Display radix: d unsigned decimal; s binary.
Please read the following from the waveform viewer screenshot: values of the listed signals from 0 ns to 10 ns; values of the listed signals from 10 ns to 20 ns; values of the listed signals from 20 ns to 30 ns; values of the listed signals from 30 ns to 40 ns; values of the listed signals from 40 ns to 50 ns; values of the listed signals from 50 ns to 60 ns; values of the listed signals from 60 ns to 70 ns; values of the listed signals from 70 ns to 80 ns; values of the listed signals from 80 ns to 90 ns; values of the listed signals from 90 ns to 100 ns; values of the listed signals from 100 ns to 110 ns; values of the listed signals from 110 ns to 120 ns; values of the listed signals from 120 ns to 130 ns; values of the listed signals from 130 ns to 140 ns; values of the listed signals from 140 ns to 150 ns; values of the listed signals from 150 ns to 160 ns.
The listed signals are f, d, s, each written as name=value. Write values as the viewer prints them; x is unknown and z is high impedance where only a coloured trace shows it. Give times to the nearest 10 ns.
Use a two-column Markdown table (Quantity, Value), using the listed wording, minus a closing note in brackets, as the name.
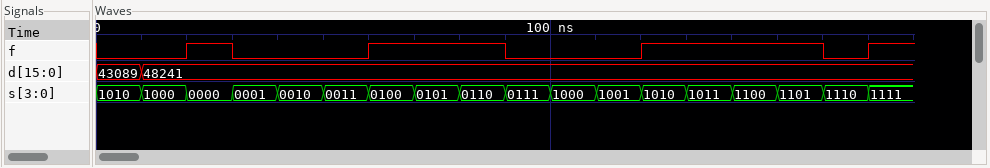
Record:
| Quantity | Value |
|---|---|
| values of the listed signals from 0 ns to 10 ns | f=0, d=43089, s=1010 |
| values of the listed signals from 10 ns to 20 ns | f=0, d=48241, s=1000 |
| values of the listed signals from 20 ns to 30 ns | f=1, d=48241, s=0000 |
| values of the listed signals from 30 ns to 40 ns | f=0, d=48241, s=0001 |
| values of the listed signals from 40 ns to 50 ns | f=0, d=48241, s=0010 |
| values of the listed signals from 50 ns to 60 ns | f=0, d=48241, s=0011 |
| values of the listed signals from 60 ns to 70 ns | f=1, d=48241, s=0100 |
| values of the listed signals from 70 ns to 80 ns | f=1, d=48241, s=0101 |
| values of the listed signals from 80 ns to 90 ns | f=1, d=48241, s=0110 |
| values of the listed signals from 90 ns to 100 ns | f=0, d=48241, s=0111 |
| values of the listed signals from 100 ns to 110 ns | f=0, d=48241, s=1000 |
| values of the listed signals from 110 ns to 120 ns | f=0, d=48241, s=1001 |
| values of the listed signals from 120 ns to 130 ns | f=1, d=48241, s=1010 |
| values of the listed signals from 130 ns to 140 ns | f=1, d=48241, s=1011 |
| values of the listed signals from 140 ns to 150 ns | f=1, d=48241, s=1100 |
| values of the listed signals from 150 ns to 160 ns | f=1, d=48241, s=1101 |
